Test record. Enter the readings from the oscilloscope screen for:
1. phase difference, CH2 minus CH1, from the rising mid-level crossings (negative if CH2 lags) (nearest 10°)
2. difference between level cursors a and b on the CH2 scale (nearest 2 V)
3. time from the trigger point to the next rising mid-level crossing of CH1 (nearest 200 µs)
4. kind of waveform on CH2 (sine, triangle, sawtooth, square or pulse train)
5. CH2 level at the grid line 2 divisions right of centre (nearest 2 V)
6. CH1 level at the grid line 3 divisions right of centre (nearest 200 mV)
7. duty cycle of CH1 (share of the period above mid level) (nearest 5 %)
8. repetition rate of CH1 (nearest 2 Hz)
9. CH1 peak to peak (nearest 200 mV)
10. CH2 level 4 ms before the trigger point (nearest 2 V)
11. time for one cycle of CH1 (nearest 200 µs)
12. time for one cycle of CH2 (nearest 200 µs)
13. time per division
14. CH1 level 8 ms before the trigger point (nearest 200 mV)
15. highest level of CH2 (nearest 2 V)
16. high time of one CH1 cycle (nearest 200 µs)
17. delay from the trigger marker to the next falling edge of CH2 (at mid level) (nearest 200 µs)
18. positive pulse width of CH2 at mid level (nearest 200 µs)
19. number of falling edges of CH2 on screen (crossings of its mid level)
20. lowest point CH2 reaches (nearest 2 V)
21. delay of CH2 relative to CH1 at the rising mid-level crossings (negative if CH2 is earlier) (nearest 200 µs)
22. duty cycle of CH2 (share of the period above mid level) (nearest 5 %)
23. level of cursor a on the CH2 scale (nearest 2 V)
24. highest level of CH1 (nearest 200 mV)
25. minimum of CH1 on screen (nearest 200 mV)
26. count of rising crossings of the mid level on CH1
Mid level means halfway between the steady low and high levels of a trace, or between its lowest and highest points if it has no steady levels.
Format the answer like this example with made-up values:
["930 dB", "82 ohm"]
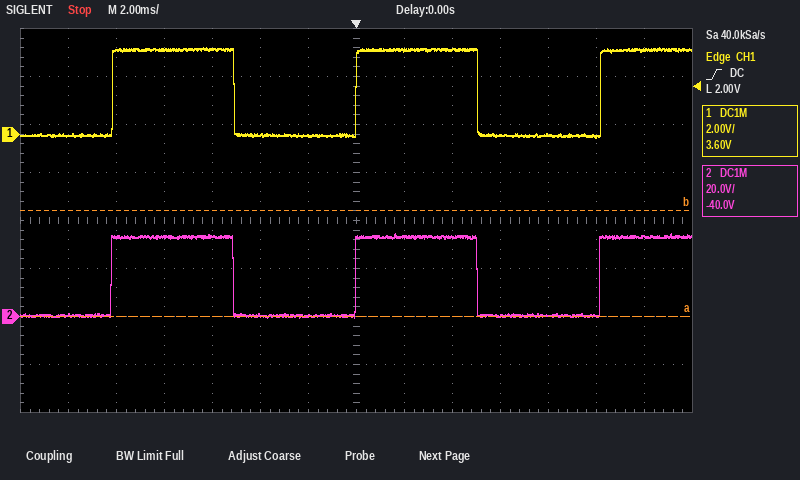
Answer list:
["0°", "44 V", "10.2 ms", "square", "34 V", "0.0 V", "50 %", "98 Hz", "3.8 V", "0 V", "10.2 ms", "10.2 ms", "2 ms", "3.6 V", "34 V", "5.0 ms", "5.0 ms", "5.0 ms", "2", "0 V", "0.0 ms", "50 %", "0 V", "3.6 V", "-200 mV", "3"]
